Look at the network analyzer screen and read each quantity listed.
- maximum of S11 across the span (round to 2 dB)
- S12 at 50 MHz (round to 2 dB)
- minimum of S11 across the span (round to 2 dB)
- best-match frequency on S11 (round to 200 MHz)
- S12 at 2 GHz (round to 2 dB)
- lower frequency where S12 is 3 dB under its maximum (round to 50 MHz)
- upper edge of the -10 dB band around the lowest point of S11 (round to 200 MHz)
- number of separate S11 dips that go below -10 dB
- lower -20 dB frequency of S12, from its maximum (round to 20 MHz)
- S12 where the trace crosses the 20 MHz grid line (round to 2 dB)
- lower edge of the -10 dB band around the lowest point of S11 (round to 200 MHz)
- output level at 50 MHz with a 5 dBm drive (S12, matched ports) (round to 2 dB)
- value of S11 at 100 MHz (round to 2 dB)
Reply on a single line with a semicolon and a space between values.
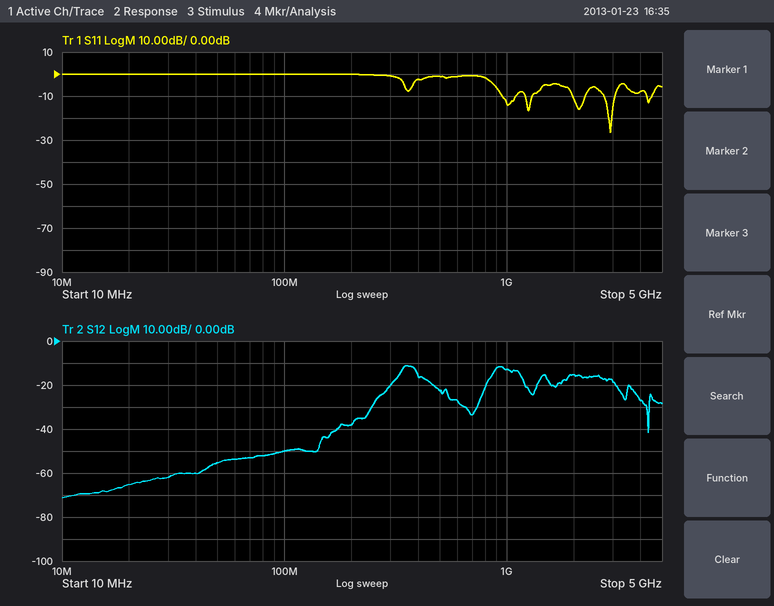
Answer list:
0 dB; -56 dB; -26 dB; 3.0 GHz; -16 dB; 350 MHz; 3.0 GHz; 5; 240 MHz; -66 dB; 2.8 GHz; -50 dBm; 0 dB
